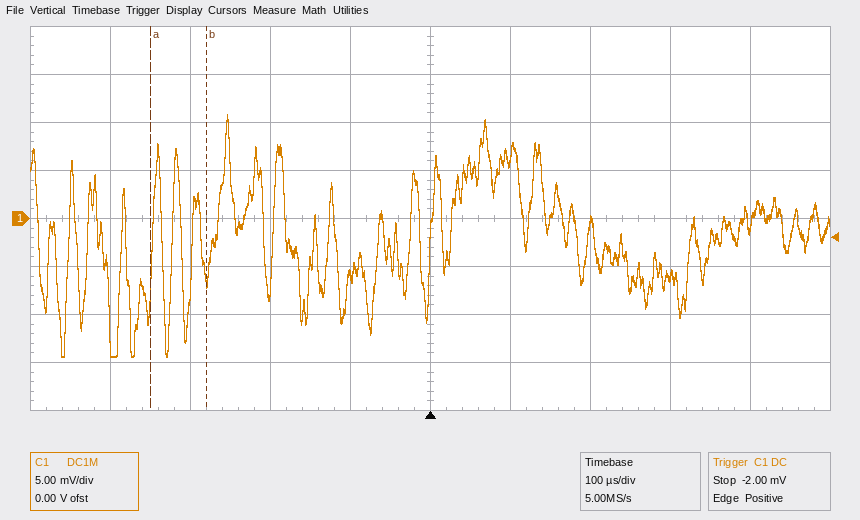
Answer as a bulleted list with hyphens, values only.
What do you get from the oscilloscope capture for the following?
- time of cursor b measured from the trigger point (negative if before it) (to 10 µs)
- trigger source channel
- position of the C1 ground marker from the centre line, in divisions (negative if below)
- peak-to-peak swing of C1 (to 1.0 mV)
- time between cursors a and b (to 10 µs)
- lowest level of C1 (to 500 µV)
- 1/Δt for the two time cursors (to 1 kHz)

- -280 µs
- C1
- 0.0 div
- 25.0 mV
- 70 µs
- -14.5 mV
- 14 kHz
